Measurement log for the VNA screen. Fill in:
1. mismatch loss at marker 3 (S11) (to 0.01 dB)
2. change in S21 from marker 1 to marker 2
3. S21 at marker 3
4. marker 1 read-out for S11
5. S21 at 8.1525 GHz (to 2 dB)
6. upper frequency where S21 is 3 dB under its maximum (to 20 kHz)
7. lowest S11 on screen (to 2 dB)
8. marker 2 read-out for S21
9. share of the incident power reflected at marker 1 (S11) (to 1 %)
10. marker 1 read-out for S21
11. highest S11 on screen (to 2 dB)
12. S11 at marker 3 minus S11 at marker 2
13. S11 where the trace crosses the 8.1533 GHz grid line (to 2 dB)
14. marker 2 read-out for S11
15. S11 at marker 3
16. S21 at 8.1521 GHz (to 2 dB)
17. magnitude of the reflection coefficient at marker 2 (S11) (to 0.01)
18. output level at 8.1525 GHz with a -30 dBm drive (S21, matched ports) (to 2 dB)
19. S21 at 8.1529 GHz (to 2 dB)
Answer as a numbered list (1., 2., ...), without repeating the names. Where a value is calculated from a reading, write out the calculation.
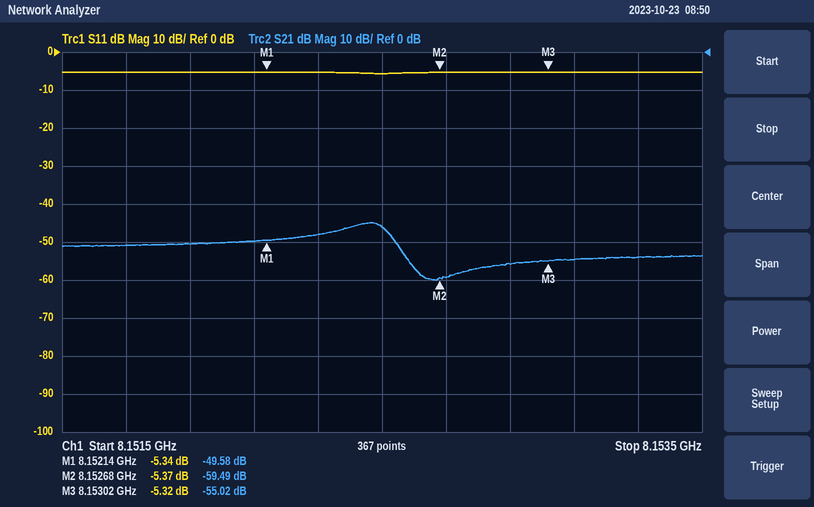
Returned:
1. −10 log10(1 − 10^(-5.32/10)) ≈ 1.51 dB
2. -59.49 − (-49.58) = -9.91 dB
3. -55.02 dB
4. -5.34 dB
5. -46 dB
6. 8.15252 GHz
7. -6 dB
8. -59.49 dB
9. 10^(-5.34/10) ≈ 29 %
10. -49.58 dB
11. -6 dB
12. -5.32 − (-5.37) = 0.05 dB
13. -6 dB
14. -5.37 dB
15. -5.32 dB
16. -50 dB
17. 10^(-5.37/20) ≈ 0.54
18. -30 dBm + (-46 dB) = -76 dBm
19. -56 dB
